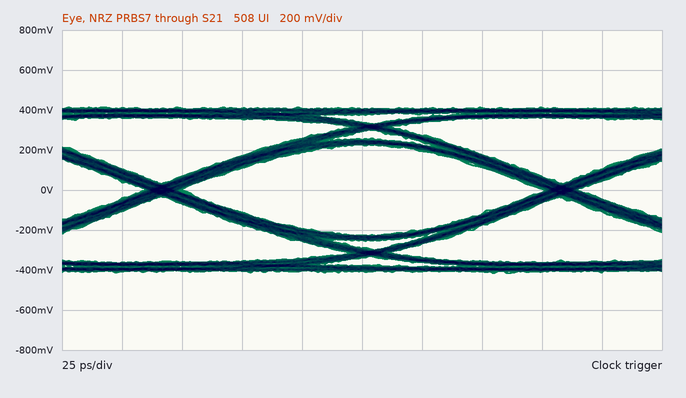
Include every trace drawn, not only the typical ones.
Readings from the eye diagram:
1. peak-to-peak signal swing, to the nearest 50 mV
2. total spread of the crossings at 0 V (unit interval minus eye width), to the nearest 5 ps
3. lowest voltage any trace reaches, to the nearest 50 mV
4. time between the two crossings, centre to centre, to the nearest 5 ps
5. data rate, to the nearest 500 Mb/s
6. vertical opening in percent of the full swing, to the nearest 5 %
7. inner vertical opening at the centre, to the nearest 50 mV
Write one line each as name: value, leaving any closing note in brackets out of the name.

peak-to-peak signal swing, to the nearest 50 mV: 850 mV
total spread of the crossings at 0 V (unit interval minus eye width), to the nearest 5 ps: 15 ps
lowest voltage any trace reaches, to the nearest 50 mV: -400 mV
time between the two crossings, centre to centre, to the nearest 5 ps: 165 ps
data rate, to the nearest 500 Mb/s: 6.0 Gb/s
vertical opening in percent of the full swing, to the nearest 5 %: 55 %
inner vertical opening at the centre, to the nearest 50 mV: 450 mV
